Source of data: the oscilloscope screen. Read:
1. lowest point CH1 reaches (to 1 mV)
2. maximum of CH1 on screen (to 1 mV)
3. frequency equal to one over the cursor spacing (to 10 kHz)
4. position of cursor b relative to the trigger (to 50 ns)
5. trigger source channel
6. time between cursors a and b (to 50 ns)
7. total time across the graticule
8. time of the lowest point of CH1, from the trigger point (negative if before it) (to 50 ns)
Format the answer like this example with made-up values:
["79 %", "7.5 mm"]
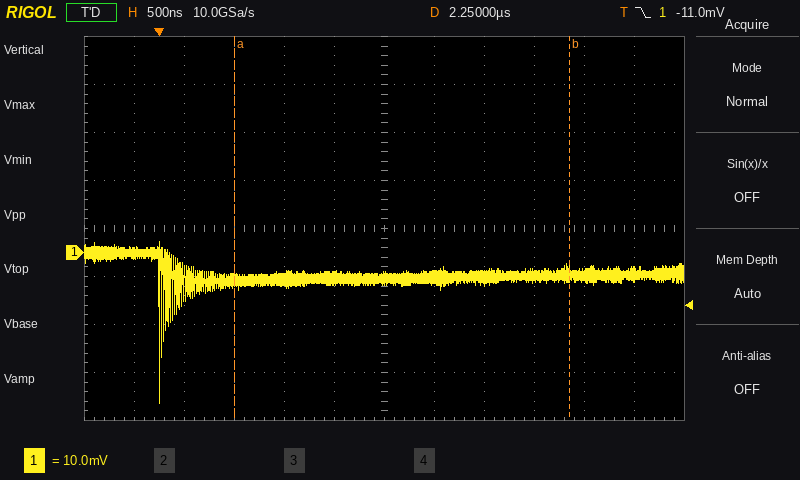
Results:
["-31 mV", "2 mV", "300 kHz", "+4.10 µs", "CH1", "3.35 µs", "6 µs", "0 ns"]
